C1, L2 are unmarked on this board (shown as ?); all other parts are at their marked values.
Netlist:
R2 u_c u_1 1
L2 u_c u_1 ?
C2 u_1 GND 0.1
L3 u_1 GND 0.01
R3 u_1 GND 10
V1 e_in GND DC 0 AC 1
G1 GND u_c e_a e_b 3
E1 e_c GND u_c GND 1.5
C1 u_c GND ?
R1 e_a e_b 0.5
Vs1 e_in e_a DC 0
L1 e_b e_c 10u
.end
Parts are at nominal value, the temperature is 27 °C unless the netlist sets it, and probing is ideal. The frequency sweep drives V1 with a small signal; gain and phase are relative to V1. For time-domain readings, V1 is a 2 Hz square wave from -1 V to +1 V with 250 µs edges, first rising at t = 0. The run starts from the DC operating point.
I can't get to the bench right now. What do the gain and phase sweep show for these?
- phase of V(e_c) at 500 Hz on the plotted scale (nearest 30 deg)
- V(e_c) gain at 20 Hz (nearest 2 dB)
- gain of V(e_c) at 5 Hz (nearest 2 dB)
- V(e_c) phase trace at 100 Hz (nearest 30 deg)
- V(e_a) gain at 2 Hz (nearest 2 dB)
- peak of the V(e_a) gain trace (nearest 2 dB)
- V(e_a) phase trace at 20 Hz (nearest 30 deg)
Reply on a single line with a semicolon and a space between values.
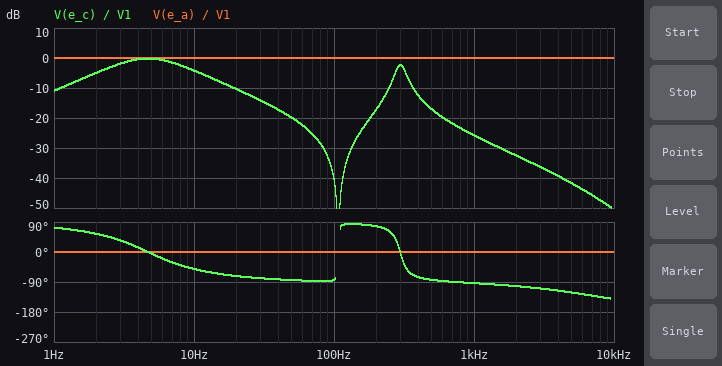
-90 deg; -10 dB; 0 dB; -90 deg; 0 dB; 0 dB; 0 deg
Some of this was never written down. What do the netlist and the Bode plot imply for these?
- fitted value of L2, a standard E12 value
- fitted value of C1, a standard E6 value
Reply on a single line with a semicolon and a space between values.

22 µH; 15 mF
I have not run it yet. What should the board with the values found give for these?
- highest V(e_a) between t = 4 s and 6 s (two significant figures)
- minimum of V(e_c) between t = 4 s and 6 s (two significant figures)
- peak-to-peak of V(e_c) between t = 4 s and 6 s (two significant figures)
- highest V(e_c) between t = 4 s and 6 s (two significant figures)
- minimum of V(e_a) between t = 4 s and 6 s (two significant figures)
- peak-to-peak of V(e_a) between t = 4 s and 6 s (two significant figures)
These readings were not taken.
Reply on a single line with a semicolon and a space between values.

1.0 V; -1.2 V; 2.5 V; 1.2 V; -1.0 V; 2.0 V
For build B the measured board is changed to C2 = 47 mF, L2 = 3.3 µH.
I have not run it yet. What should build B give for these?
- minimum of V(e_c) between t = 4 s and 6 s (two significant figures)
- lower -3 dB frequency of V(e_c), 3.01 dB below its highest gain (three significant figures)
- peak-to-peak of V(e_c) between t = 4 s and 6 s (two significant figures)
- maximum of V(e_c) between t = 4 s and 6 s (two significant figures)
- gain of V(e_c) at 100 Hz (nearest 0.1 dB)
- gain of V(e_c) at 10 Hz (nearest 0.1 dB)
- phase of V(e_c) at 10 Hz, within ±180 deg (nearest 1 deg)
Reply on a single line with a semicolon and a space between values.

-1.4 V; 2.80 Hz; 2.8 V; 1.4 V; -19.2 dB; -1.2 dB; -27 deg
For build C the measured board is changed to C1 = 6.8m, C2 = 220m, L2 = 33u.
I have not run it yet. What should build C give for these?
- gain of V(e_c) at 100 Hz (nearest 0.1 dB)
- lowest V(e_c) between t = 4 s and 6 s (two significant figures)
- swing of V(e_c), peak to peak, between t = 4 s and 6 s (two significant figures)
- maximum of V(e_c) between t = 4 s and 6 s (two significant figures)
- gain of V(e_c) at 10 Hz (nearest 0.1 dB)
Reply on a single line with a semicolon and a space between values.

-23.9 dB; -1.1 V; 2.2 V; 1.1 V; -9.7 dB
